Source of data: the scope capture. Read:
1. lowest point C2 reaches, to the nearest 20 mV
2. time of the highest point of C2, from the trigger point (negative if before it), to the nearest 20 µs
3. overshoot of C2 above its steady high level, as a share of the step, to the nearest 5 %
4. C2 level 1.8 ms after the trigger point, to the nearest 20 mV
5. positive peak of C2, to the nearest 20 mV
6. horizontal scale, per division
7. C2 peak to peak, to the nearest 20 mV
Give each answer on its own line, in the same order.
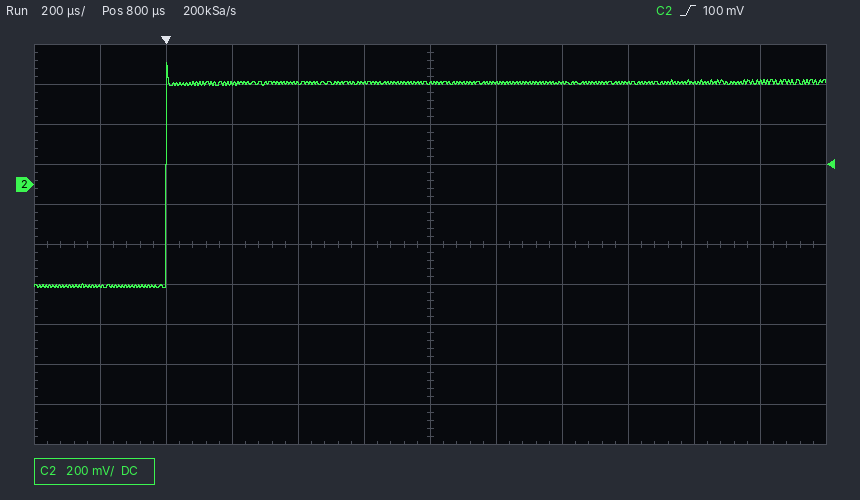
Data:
-520 mV
0 µs
10 %
520 mV
600 mV
200 µs
1.12 V
